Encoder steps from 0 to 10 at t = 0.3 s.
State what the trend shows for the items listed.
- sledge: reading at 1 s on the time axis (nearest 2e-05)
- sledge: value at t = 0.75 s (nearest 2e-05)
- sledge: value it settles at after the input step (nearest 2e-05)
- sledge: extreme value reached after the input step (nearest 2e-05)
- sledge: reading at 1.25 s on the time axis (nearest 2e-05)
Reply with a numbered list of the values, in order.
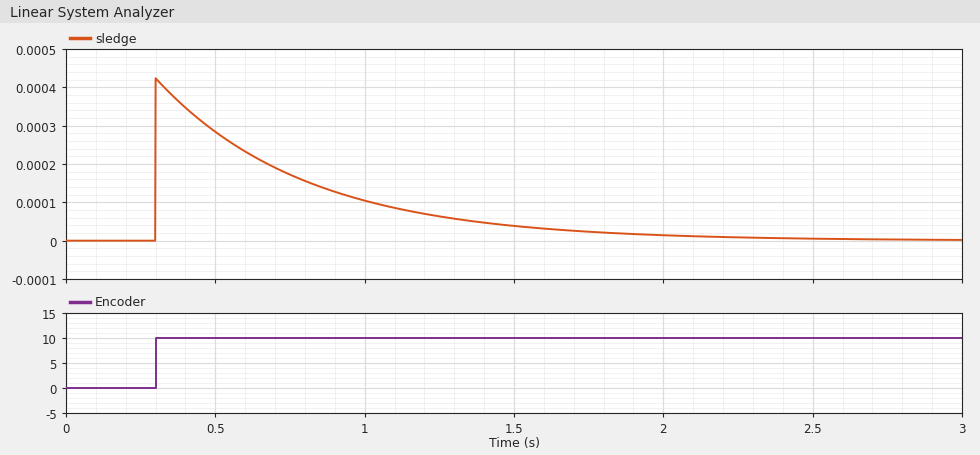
1. 0.00010
2. 0.00018
3. 0.00000
4. 0.00042
5. 0.00006
